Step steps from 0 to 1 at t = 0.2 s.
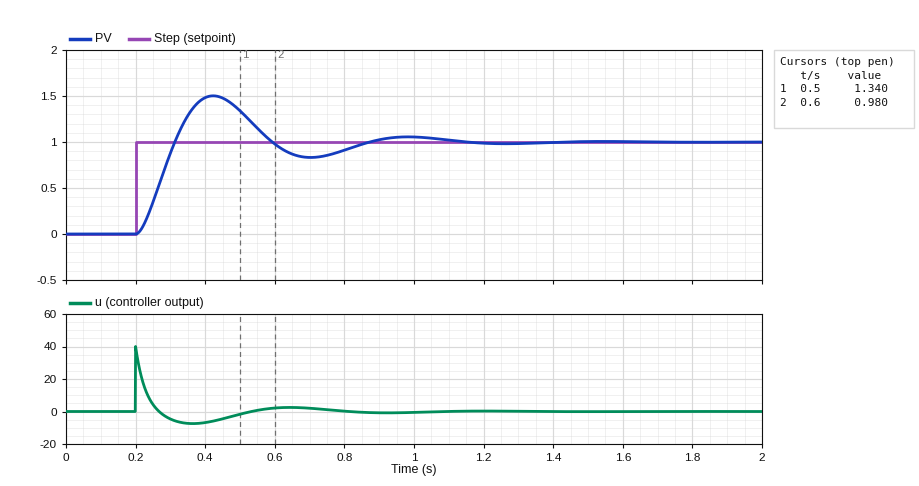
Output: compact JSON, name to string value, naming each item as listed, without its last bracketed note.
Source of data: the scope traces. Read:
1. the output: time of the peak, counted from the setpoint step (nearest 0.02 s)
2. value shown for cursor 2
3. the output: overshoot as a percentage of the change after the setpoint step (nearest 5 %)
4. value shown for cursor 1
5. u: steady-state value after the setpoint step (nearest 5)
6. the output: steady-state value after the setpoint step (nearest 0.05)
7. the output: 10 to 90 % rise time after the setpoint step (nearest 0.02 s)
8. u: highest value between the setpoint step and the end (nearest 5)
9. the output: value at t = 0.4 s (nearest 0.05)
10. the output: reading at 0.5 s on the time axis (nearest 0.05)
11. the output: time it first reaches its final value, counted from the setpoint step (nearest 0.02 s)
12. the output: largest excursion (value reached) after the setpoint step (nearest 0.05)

{"the output: time of the peak, counted from the setpoint step": "0.22 s", "value shown for cursor 2": "0.980", "the output: overshoot as a percentage of the change after the setpoint step": "50 %", "value shown for cursor 1": "1.340", "u: steady-state value after the setpoint step": "0", "the output: steady-state value after the setpoint step": "1.00", "the output: 10 to 90 % rise time after the setpoint step": "0.08 s", "u: highest value between the setpoint step and the end": "40", "the output: value at t = 0.4 s": "1.50", "the output: reading at 0.5 s on the time axis": "1.35", "the output: time it first reaches its final value, counted from the setpoint step": "0.12 s", "the output: largest excursion (value reached) after the setpoint step": "1.50"}
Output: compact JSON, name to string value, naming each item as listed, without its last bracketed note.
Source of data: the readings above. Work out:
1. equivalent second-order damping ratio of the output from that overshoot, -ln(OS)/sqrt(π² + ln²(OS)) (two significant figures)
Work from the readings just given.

{"equivalent second-order damping ratio of the output from that overshoot, -ln(OS)/sqrt(π² + ln²(OS))": "0.22"}
